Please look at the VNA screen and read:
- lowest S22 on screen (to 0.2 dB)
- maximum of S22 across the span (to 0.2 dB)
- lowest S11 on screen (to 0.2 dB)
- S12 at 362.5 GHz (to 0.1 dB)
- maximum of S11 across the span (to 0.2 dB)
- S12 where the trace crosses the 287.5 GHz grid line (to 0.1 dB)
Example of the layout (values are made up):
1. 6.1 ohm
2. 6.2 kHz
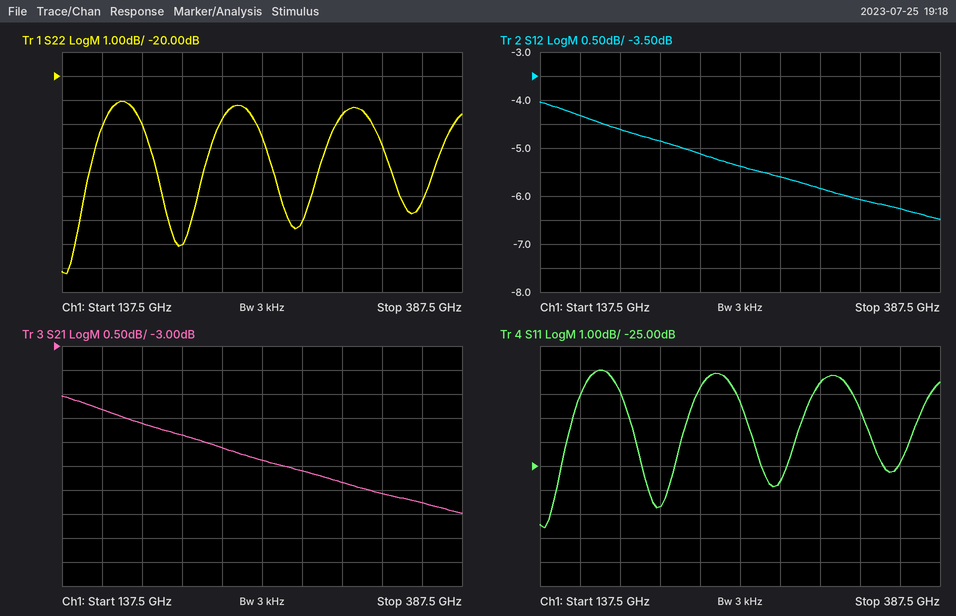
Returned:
1. -28.2 dB
2. -21.0 dB
3. -27.6 dB
4. -6.3 dB
5. -21.0 dB
6. -5.6 dB
